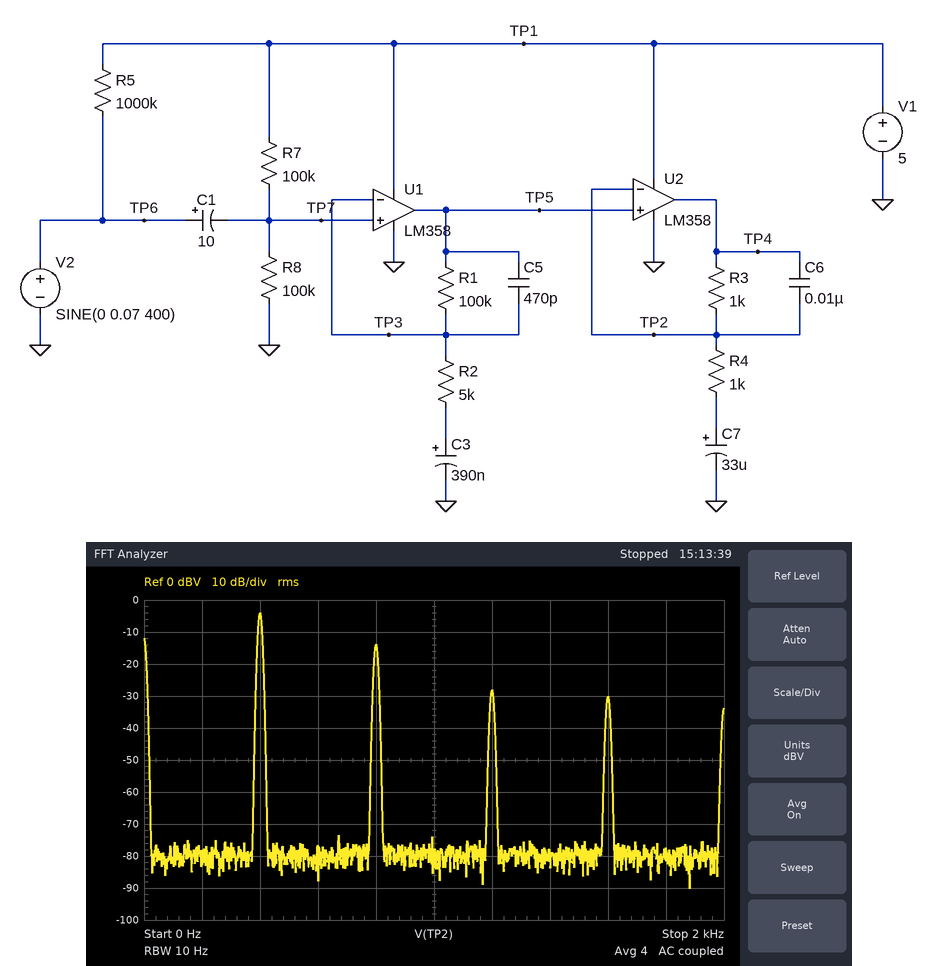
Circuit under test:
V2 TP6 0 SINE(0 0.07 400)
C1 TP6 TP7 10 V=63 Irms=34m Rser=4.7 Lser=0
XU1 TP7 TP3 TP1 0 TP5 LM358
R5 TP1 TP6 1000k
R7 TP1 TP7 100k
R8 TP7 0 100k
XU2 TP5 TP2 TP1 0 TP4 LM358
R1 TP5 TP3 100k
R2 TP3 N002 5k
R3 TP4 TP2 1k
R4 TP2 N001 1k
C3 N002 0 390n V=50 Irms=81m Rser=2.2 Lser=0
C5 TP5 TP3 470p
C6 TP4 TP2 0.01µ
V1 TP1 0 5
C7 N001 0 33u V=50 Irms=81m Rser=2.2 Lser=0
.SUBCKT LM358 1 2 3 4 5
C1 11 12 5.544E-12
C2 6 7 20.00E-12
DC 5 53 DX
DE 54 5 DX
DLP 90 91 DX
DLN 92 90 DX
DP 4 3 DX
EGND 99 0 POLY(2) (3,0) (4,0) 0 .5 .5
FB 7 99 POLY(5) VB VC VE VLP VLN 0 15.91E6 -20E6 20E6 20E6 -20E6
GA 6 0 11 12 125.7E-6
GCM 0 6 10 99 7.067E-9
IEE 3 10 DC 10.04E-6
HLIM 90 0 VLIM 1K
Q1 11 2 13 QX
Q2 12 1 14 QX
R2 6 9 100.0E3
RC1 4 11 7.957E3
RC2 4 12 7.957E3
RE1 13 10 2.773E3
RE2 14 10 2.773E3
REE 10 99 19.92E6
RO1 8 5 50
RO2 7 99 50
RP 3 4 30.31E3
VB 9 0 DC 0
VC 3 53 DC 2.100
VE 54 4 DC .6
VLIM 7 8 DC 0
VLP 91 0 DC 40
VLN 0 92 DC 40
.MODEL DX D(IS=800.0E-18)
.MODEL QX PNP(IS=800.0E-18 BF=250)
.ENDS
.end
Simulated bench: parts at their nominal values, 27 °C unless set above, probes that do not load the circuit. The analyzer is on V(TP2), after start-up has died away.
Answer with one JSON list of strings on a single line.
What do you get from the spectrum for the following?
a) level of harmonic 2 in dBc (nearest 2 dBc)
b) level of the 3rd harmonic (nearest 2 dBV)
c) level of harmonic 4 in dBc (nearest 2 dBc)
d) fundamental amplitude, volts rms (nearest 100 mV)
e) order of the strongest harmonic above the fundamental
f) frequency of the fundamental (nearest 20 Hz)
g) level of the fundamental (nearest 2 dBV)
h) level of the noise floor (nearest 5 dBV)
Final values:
["-10 dBc", "-28 dBV", "-26 dBc", "600 mV", "2", "400 Hz", "-4 dBV", "-80 dBV"]
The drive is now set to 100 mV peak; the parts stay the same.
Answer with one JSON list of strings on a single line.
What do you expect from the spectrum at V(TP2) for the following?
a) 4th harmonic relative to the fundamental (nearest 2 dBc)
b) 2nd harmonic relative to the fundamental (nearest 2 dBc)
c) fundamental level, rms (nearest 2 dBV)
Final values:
["-18 dBc", "-8 dBc", "-4 dBV"]
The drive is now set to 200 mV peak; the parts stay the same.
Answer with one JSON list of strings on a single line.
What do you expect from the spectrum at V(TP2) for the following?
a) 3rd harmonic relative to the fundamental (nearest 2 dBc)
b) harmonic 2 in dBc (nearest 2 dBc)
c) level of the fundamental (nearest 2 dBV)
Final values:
["-32 dBc", "-6 dBc", "-4 dBV"]
